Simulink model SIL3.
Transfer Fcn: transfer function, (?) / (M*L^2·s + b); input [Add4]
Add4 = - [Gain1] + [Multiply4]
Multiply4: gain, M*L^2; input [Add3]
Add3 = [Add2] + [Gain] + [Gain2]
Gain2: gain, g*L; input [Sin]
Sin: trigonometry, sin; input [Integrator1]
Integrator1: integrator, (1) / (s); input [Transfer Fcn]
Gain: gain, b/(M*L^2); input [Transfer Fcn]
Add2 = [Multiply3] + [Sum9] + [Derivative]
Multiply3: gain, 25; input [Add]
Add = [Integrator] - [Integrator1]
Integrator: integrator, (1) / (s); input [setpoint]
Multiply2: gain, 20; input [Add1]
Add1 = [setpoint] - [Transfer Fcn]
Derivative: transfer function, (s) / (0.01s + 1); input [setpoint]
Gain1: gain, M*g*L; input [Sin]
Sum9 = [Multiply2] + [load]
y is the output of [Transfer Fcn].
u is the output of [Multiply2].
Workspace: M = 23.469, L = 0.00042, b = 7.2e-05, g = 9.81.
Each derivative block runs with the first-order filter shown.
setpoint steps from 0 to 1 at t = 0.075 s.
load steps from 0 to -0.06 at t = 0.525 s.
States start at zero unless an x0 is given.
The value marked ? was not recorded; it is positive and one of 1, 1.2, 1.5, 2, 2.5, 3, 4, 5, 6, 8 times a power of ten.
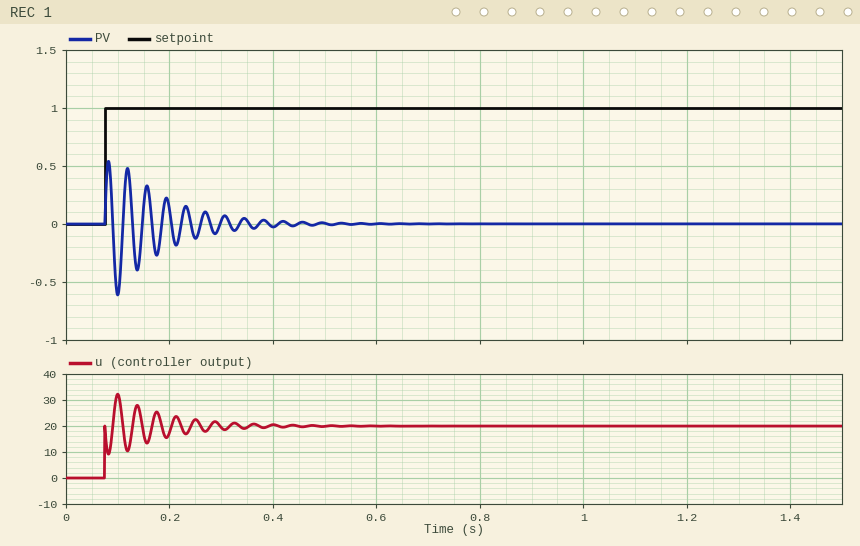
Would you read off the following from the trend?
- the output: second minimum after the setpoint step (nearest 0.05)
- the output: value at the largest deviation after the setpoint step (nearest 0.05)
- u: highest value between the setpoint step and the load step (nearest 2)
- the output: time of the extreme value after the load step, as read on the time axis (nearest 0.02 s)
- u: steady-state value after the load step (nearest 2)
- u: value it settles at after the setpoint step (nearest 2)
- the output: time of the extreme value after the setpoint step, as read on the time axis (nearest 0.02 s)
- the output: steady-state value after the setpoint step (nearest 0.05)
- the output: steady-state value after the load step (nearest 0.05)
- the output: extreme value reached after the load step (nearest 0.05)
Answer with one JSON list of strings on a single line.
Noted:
["-0.40", "-0.60", "32", "0.54 s", "20", "20", "0.10 s", "0.00", "0.00", "0.00"]
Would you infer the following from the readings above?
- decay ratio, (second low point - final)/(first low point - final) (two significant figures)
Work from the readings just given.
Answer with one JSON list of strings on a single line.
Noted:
["0.67"]
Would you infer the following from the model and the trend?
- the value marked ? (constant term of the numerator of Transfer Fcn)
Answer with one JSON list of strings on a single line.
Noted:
["1.2"]
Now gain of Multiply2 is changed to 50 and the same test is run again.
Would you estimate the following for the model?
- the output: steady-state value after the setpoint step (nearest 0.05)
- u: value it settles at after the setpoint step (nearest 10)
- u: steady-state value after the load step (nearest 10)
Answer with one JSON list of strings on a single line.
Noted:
["0.00", "50", "50"]
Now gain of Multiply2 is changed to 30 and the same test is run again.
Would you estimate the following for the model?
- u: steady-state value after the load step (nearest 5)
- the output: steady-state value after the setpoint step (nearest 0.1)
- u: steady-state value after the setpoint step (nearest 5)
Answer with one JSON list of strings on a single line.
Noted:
["30", "0.0", "30"]
